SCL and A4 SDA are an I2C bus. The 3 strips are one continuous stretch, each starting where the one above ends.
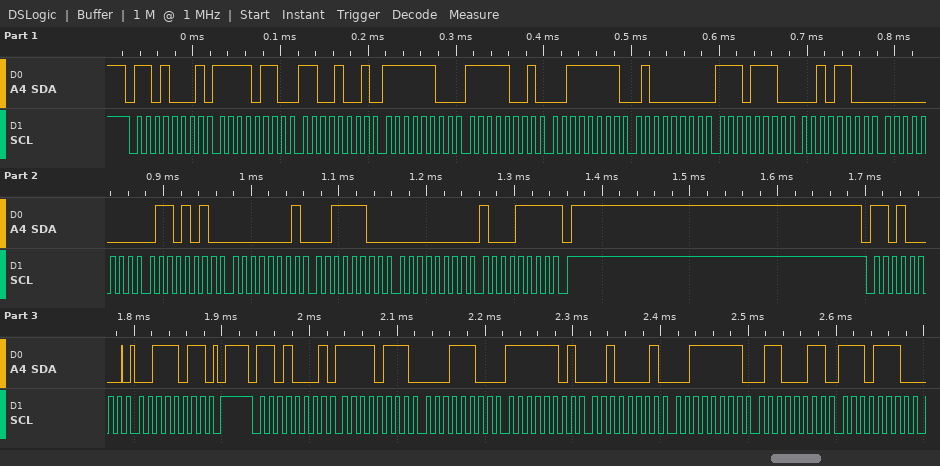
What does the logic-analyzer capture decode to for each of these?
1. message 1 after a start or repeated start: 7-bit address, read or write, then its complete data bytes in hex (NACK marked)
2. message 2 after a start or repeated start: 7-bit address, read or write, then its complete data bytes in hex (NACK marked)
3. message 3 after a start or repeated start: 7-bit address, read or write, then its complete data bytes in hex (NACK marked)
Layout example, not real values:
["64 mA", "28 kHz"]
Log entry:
["0x68 read: F6 C9 FC F9 3F 40 EE 2C 00 6A 01 3C 00 8F NACK", "0x68 write: 3B", "0x68 read: F7 1C FD 21 3F 63 EE"]
